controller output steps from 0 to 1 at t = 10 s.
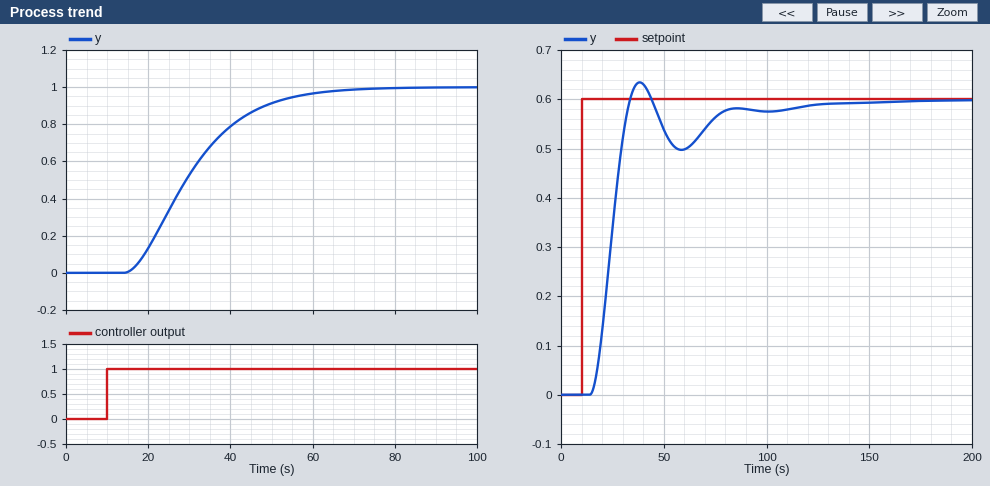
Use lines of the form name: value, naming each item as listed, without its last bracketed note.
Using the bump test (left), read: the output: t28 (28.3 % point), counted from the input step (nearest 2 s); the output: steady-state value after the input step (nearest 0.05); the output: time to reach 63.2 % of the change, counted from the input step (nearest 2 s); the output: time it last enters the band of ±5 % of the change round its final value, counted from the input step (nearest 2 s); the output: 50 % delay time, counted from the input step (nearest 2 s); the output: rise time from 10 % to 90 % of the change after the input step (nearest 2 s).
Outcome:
the output: t28 (28.3 % point), counted from the input step: 14 s
the output: steady-state value after the input step: 1.00
the output: time to reach 63.2 % of the change, counted from the input step: 24 s
the output: time it last enters the band of ±5 % of the change round its final value, counted from the input step: 46 s
the output: 50 % delay time, counted from the input step: 20 s
the output: rise time from 10 % to 90 % of the change after the input step: 30 s
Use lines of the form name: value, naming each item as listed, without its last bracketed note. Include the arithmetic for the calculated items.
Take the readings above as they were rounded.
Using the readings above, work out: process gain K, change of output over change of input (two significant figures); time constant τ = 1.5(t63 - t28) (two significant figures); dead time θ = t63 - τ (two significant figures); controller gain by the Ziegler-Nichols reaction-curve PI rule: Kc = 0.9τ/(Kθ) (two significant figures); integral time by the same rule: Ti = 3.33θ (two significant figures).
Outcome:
process gain K, change of output over change of input: (1 - 0) / 1 = 1.0
time constant τ = 1.5(t63 - t28): 1.5 × (24 - 14) = 15 s
dead time θ = t63 - τ: 24 - 15 = 9.0 s
controller gain by the Ziegler-Nichols reaction-curve PI rule: Kc = 0.9τ/(Kθ): 0.9 × 15 / (1 × 9) = 1.5
integral time by the same rule: Ti = 3.33θ: 3.33 × 9 = 30 s
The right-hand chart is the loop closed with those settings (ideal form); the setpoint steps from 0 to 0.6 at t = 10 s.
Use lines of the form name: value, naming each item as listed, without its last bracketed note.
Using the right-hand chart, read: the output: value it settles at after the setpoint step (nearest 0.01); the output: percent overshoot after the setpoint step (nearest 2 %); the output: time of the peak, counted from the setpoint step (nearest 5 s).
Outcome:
the output: value it settles at after the setpoint step: 0.60
the output: percent overshoot after the setpoint step: 6 %
the output: time of the peak, counted from the setpoint step: 30 s
